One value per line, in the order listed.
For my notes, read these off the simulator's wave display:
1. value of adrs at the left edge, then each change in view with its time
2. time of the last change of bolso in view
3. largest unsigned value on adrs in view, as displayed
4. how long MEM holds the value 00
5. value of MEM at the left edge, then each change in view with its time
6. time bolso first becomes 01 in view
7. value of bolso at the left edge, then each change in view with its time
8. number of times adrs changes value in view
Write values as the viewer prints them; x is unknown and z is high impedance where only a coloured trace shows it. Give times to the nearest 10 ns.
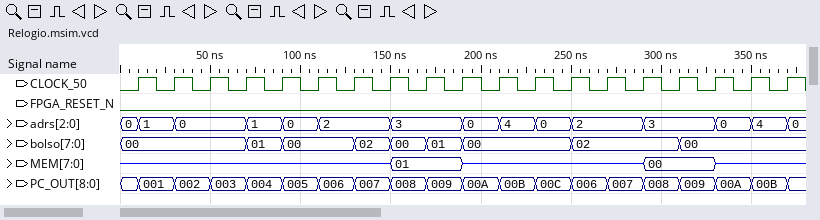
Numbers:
0, 1 at 10 ns, 0 at 30 ns, 1 at 70 ns, 0 at 90 ns, 2 at 110 ns, 3 at 150 ns, 0 at 190 ns, 4 at 210 ns, 0 at 230 ns, 2 at 250 ns, 3 at 290 ns, 0 at 330 ns, 4 at 350 ns, 0 at 370 ns
310 ns
4
40 ns
z, 01 at 150 ns, z at 190 ns, 00 at 290 ns, z at 330 ns
70 ns
00, 01 at 70 ns, 00 at 90 ns, 02 at 130 ns, 00 at 150 ns, 01 at 170 ns, 00 at 190 ns, 02 at 250 ns, 00 at 310 ns
14
